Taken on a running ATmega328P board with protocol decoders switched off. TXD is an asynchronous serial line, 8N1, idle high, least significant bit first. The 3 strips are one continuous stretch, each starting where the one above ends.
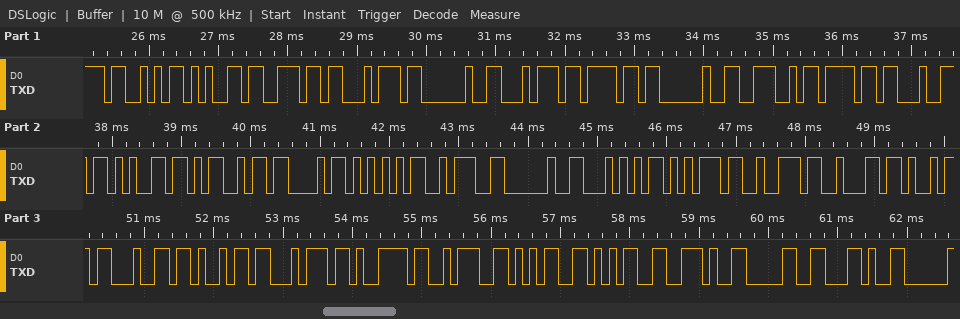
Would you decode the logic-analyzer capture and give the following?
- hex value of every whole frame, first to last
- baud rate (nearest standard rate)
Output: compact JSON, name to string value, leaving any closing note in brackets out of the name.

{"hex value of every whole frame, first to last": "53 65 6E 74 20 74 6F 20 4E 6F 64 65 4D 43 55 3A 20 54 75 72 62 69 64 69 74 79 3A 35 35 2E 30 2C", "baud rate": "9600 baud"}
